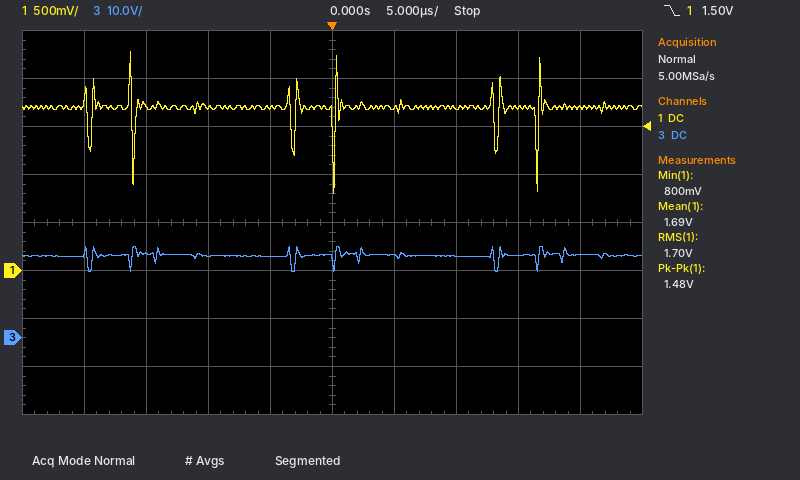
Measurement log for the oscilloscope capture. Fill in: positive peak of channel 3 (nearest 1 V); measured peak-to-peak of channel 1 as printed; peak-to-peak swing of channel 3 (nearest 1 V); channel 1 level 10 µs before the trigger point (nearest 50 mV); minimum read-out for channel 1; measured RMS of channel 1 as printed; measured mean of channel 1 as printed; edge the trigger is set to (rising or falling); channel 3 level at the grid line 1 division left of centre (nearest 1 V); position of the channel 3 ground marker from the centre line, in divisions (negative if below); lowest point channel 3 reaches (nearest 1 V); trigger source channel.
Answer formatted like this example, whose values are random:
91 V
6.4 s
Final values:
19 V
1.48 V
5 V
1.70 V
800 mV
1.70 V
1.69 V
falling
17 V
-2.4 div
14 V
channel 1
